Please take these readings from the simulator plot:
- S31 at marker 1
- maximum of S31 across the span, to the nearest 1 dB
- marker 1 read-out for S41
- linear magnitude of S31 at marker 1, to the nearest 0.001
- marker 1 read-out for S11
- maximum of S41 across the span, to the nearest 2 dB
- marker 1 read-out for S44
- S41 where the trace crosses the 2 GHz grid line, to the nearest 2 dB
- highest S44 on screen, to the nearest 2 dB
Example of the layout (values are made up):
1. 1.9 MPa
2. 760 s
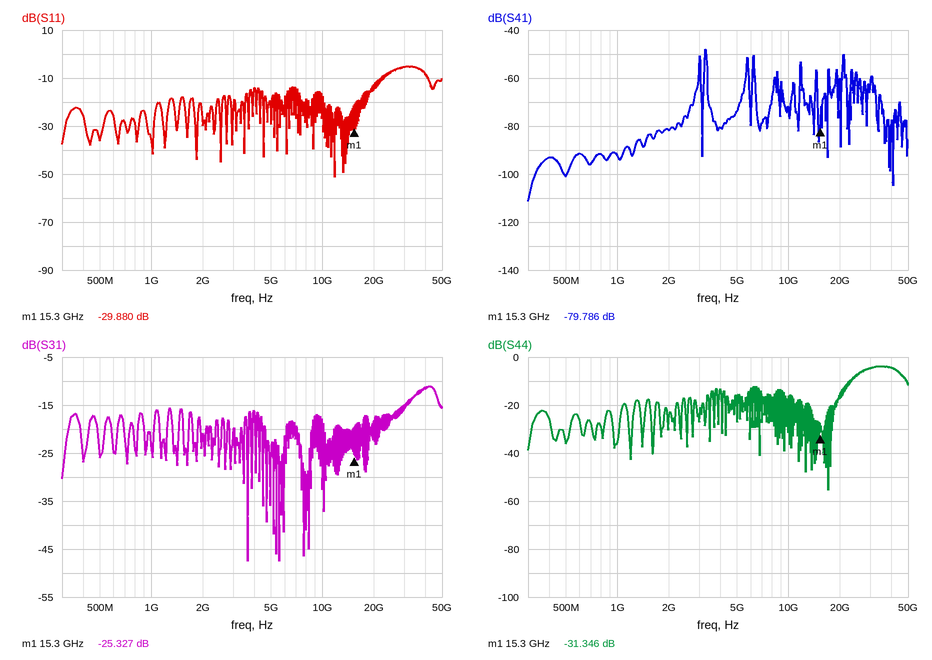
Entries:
1. -25.327 dB
2. -11 dB
3. -79.786 dB
4. 0.054
5. -29.880 dB
6. -48 dB
7. -31.346 dB
8. -82 dB
9. -4 dB
